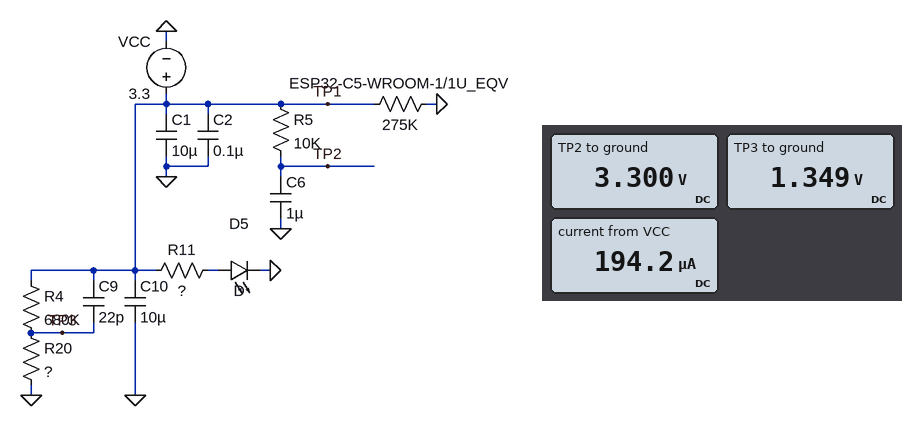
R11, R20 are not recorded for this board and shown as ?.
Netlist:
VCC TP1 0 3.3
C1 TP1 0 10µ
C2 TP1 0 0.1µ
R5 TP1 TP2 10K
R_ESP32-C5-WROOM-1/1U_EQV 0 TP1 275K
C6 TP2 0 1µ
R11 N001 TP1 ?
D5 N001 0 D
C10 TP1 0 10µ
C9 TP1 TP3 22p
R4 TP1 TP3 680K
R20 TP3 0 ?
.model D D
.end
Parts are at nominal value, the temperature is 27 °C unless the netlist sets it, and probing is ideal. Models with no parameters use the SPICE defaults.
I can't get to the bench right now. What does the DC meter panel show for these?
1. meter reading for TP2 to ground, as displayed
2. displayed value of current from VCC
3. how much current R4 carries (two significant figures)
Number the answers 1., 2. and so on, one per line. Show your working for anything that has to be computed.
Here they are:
1. 3.300 V
2. 194.2 µA
3. (3.3 V - 1.349 V) / 680 kΩ = 2.9 µA
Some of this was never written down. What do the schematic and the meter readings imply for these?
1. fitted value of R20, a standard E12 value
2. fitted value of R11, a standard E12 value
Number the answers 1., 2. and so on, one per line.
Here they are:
1. 470 kΩ
2. 15 kΩ
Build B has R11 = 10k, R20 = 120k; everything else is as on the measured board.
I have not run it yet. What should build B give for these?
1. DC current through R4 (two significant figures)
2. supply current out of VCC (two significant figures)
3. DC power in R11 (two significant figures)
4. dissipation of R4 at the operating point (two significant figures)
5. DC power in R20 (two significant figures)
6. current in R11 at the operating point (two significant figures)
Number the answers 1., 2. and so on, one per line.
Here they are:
1. 4.1 µA
2. 280 µA
3. 720 µW
4. 12 µW
5. 2.0 µW
6. 270 µA
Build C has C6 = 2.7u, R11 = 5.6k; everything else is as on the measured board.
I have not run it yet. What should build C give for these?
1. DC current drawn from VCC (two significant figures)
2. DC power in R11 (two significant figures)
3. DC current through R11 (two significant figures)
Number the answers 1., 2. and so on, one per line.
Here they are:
1. 490 µA
2. 1.3 mW
3. 480 µA
